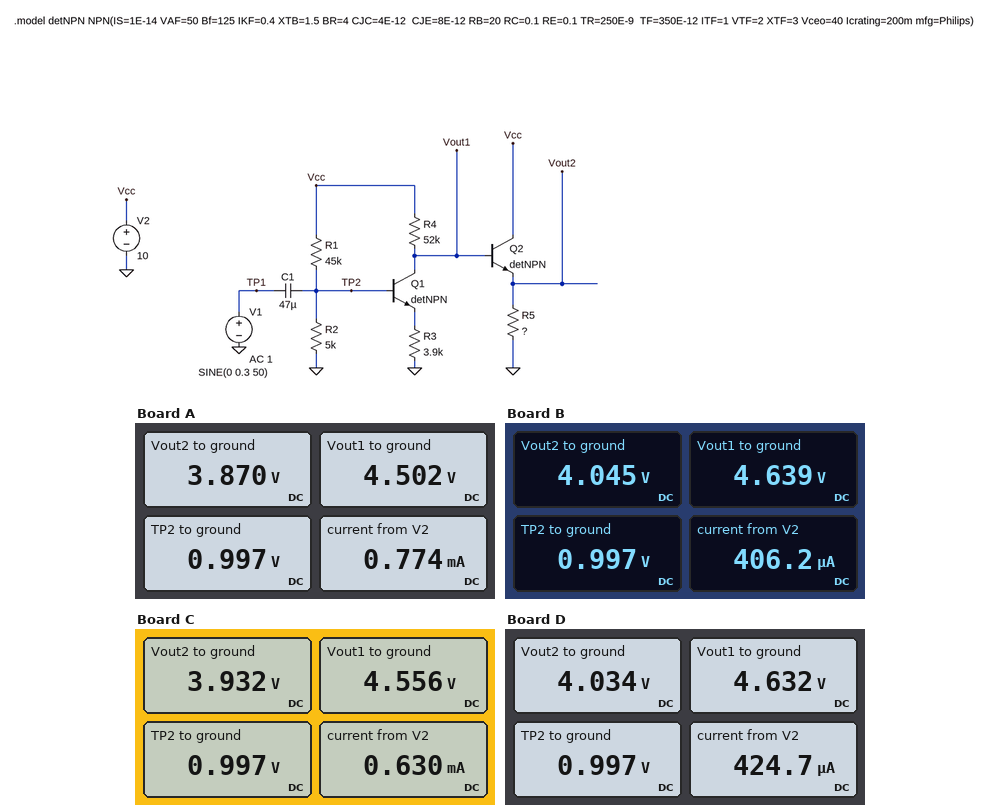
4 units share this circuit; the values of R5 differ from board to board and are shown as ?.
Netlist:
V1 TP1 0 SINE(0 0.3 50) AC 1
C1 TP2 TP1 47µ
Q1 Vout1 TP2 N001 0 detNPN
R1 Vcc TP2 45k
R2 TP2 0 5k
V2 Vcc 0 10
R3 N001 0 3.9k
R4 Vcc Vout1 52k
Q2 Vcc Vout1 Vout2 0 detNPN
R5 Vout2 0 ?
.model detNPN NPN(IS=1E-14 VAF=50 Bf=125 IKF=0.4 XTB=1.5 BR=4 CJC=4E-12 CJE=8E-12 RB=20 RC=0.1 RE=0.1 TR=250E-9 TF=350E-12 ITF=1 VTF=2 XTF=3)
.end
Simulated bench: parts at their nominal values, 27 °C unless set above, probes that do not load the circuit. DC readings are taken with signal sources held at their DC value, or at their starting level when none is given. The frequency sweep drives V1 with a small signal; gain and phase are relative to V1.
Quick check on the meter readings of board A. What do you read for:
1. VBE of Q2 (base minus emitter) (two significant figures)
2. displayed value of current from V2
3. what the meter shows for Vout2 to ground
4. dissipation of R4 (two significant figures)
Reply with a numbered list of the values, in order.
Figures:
1. 630 mV
2. 0.774 mA
3. 3.870 V
4. 580 µW
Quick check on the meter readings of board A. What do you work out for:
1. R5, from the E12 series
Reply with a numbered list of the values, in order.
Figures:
1. 8.2 kΩ
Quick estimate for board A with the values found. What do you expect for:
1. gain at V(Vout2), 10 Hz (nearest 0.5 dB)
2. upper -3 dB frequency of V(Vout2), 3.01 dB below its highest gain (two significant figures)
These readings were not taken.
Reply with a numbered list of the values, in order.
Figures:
1. 21.5 dB
2. 740 kHz
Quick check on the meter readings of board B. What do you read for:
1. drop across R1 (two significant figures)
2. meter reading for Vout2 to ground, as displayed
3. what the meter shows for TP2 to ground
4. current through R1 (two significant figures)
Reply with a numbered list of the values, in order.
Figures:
1. 9.0 V
2. 4.045 V
3. 0.997 V
4. 200 µA
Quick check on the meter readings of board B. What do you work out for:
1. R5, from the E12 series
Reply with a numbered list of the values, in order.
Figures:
1. 39 kΩ
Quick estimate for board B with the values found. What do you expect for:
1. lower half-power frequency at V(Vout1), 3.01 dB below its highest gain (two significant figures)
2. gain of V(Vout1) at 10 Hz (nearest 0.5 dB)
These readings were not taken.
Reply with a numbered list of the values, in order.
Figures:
1. 760 mHz
2. 21.5 dB
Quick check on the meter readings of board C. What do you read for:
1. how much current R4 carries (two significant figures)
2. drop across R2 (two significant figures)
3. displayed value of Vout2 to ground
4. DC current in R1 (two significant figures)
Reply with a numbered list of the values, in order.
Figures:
1. 100 µA
2. 1.0 V
3. 3.932 V
4. 200 µA
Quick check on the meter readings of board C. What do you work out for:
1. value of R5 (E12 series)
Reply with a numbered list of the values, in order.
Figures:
1. 12 kΩ
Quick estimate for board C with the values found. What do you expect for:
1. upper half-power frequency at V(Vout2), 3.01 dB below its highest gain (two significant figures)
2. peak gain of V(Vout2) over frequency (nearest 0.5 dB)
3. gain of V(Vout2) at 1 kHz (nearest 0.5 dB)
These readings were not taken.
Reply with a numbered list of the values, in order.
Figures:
1. 730 kHz
2. 21.5 dB
3. 21.5 dB
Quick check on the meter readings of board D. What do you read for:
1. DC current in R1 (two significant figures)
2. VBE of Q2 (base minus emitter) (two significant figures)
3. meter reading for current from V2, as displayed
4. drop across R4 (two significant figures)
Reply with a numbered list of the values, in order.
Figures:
1. 200 µA
2. 600 mV
3. 424.7 µA
4. 5.4 V
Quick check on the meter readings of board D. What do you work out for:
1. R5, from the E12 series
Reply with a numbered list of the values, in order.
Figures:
1. 33 kΩ
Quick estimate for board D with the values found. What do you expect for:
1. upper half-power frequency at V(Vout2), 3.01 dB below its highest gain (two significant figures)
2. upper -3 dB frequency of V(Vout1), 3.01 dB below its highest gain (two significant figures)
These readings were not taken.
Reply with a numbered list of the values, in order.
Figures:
1. 720 kHz
2. 720 kHz
